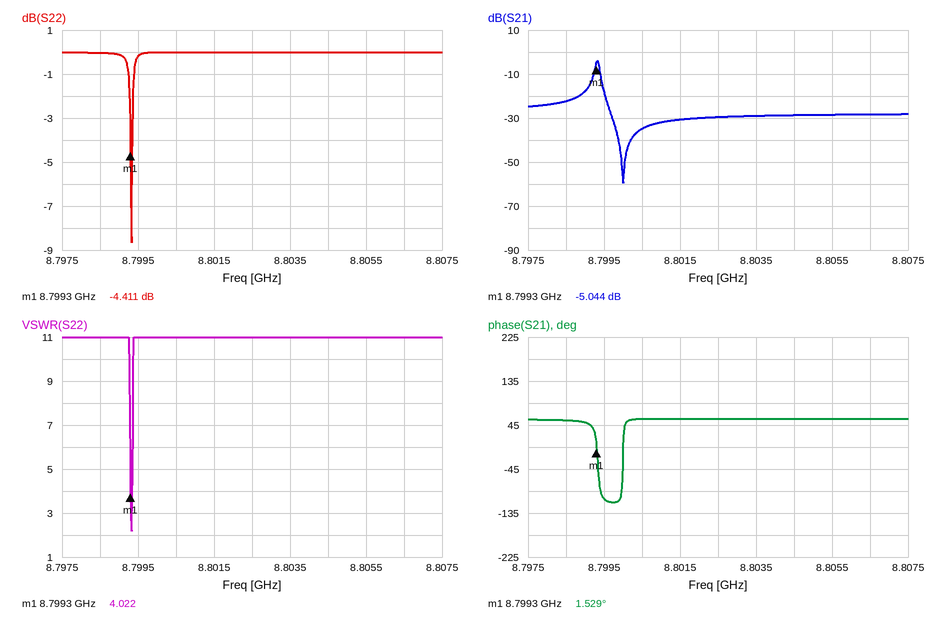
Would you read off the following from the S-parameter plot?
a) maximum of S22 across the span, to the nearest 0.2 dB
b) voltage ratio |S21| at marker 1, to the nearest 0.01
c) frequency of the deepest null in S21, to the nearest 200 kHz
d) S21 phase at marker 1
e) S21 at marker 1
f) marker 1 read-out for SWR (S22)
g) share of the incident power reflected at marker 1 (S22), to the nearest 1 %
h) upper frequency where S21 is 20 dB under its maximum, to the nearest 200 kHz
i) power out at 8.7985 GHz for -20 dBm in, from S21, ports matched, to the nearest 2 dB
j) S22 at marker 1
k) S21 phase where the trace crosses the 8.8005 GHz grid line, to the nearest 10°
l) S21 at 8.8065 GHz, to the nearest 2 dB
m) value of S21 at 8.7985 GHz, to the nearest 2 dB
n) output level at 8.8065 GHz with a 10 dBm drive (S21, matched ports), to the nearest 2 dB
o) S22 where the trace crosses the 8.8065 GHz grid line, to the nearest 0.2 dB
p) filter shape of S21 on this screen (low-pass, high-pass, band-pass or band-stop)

0.0 dB
0.56
8.8000 GHz
1.529°
-5.044 dB
4.022
36 %
8.7996 GHz
-42 dBm
-4.411 dB
60°
-28 dB
-22 dB
-18 dBm
0.0 dB
band-pass
